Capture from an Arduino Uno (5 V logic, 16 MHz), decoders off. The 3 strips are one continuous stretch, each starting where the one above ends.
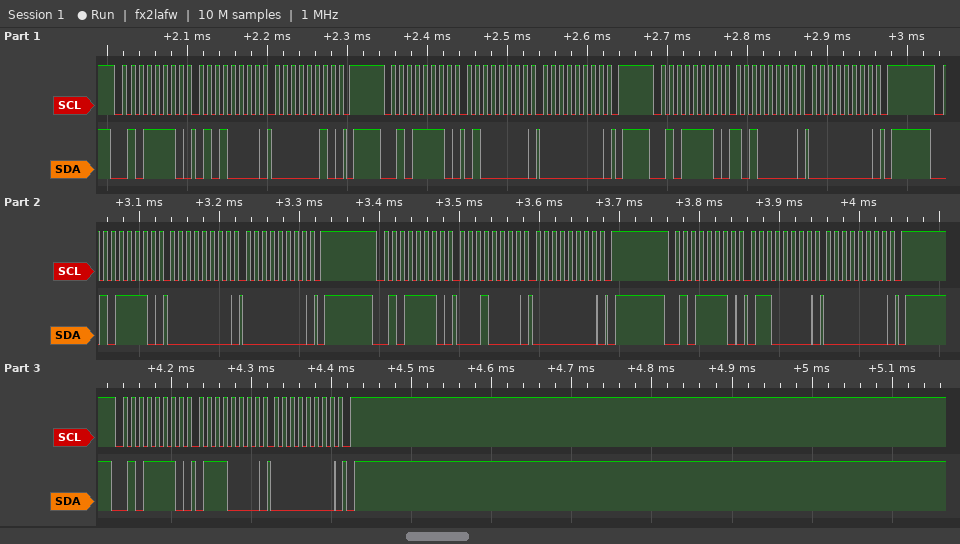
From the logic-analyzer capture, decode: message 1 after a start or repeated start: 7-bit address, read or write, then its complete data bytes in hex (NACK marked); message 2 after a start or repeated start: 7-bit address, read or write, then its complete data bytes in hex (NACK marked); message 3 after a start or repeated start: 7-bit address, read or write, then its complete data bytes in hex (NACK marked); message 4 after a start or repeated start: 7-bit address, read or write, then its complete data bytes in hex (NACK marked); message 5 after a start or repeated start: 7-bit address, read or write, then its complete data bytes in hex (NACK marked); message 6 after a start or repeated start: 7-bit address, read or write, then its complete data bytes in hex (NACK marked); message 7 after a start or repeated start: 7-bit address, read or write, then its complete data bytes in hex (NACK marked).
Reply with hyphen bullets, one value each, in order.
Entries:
- 0x2F write: 50 02
- 0x2F write: 40 00
- 0x2F write: A0 00
- 0x2F write: 00 00
- 0x2F write: 10 00
- 0x2F write: 60 00
- 0x2F write: 70 00
